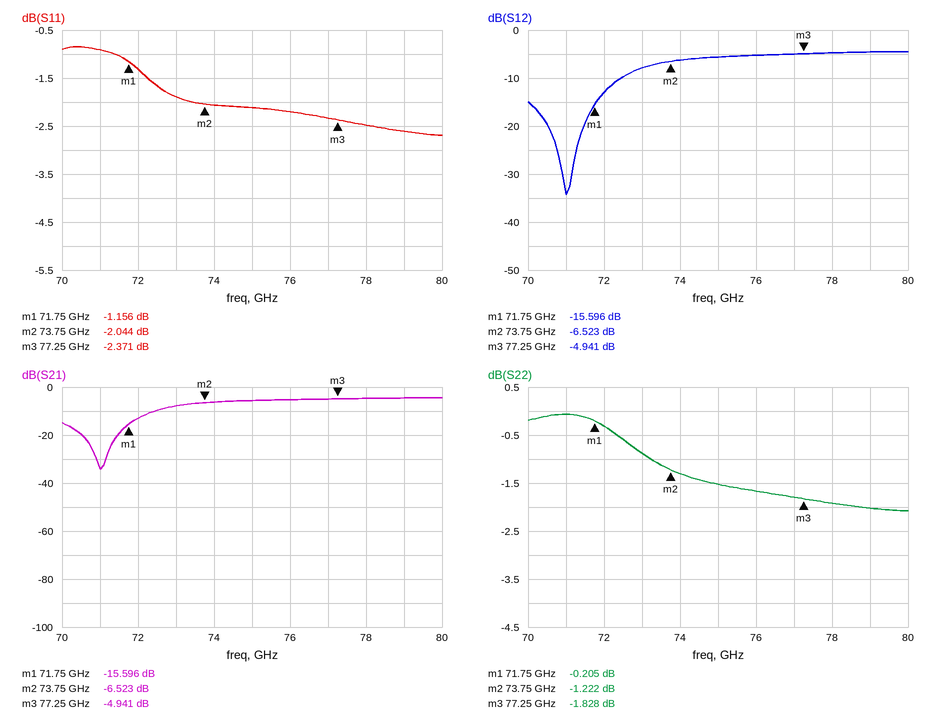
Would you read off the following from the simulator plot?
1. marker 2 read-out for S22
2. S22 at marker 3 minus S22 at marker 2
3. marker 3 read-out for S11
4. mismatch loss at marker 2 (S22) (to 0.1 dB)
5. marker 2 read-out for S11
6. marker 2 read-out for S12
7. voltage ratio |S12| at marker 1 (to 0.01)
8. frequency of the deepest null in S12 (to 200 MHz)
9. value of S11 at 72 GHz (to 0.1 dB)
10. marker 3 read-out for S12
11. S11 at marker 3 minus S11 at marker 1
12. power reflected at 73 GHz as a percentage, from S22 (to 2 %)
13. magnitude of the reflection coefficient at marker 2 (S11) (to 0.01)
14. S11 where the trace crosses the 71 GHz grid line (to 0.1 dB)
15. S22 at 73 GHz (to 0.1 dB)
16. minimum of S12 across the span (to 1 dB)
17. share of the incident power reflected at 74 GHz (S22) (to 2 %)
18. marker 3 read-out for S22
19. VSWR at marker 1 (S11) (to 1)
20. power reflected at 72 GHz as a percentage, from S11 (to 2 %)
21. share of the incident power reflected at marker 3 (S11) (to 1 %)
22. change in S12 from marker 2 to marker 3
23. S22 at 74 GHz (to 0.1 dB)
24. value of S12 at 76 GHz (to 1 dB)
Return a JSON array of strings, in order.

["-1.222 dB", "-0.606 dB", "-2.371 dB", "6.1 dB", "-2.044 dB", "-6.523 dB", "0.17", "71.0 GHz", "-1.3 dB", "-4.941 dB", "-1.215 dB", "82 %", "0.79", "-0.9 dB", "-0.9 dB", "-34 dB", "74 %", "-1.828 dB", "15", "74 %", "58 %", "1.582 dB", "-1.3 dB", "-5 dB"]
